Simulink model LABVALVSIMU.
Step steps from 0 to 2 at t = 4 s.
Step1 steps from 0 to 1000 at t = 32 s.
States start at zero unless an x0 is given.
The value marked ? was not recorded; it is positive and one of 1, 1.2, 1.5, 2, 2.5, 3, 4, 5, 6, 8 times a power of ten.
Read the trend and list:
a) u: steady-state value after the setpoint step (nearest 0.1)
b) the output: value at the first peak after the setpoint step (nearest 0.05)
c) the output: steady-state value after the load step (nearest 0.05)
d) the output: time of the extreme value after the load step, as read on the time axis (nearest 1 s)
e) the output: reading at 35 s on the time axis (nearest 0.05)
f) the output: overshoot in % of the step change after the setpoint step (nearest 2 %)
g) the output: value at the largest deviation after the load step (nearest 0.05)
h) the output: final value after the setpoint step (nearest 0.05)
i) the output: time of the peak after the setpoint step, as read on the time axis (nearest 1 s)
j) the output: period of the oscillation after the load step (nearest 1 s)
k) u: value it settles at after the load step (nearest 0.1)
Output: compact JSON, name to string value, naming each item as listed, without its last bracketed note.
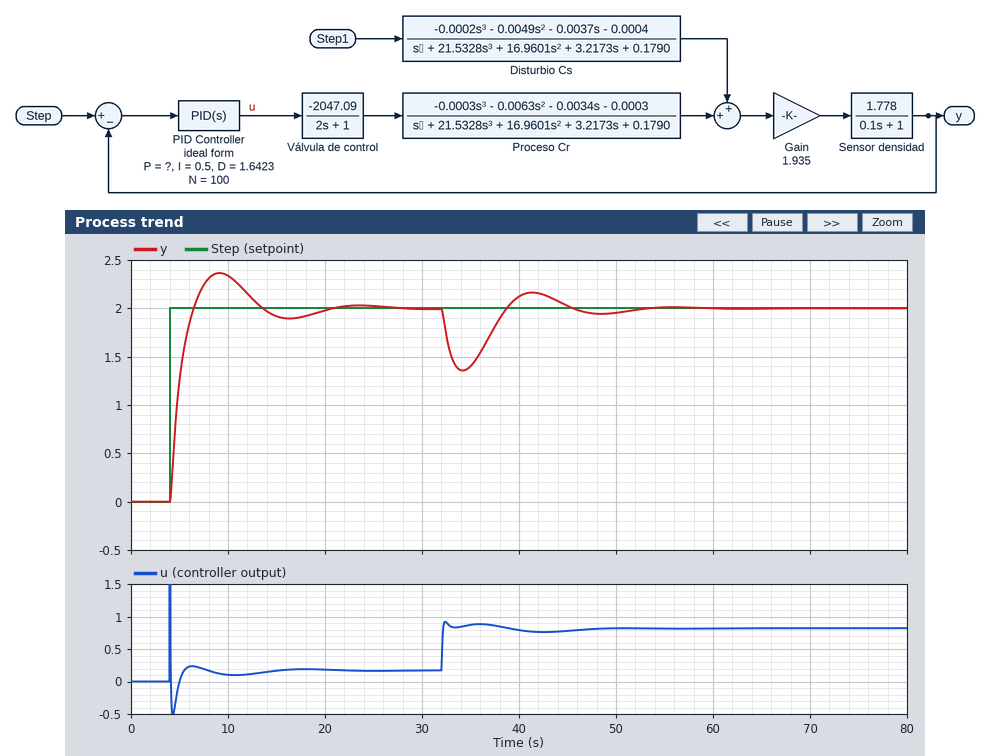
{"u: steady-state value after the setpoint step": "0.2", "the output: value at the first peak after the setpoint step": "2.35", "the output: steady-state value after the load step": "2.00", "the output: time of the extreme value after the load step, as read on the time axis": "34 s", "the output: reading at 35 s on the time axis": "1.40", "the output: overshoot in % of the step change after the setpoint step": "18 %", "the output: value at the largest deviation after the load step": "1.35", "the output: final value after the setpoint step": "2.00", "the output: time of the peak after the setpoint step, as read on the time axis": "9 s", "the output: period of the oscillation after the load step": "14 s", "u: value it settles at after the load step": "0.8"}
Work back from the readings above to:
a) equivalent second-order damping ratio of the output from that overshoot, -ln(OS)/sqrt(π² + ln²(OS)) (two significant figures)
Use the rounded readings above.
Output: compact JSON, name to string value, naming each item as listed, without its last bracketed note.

{"equivalent second-order damping ratio of the output from that overshoot, -ln(OS)/sqrt(π² + ln²(OS))": "0.48"}
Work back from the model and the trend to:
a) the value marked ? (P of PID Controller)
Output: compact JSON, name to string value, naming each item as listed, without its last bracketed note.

{"the value marked ?": "0.6"}
